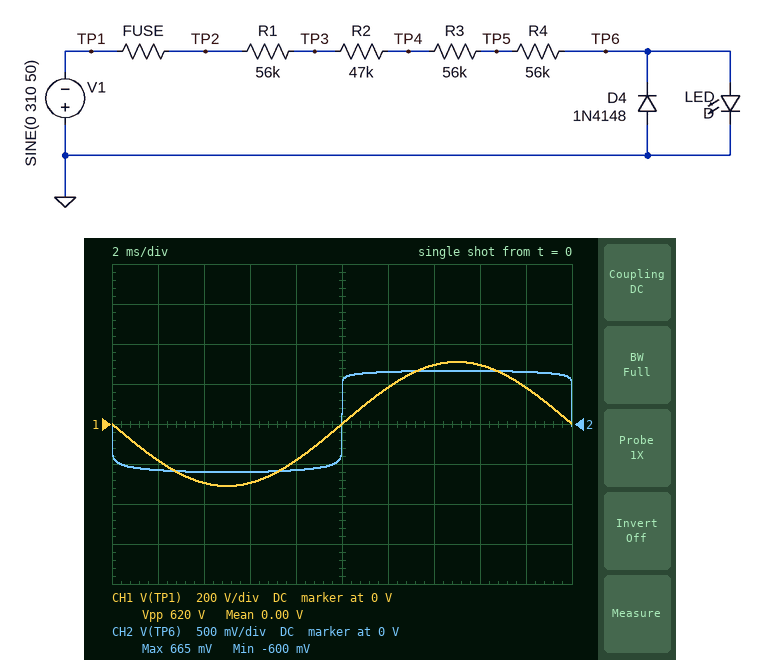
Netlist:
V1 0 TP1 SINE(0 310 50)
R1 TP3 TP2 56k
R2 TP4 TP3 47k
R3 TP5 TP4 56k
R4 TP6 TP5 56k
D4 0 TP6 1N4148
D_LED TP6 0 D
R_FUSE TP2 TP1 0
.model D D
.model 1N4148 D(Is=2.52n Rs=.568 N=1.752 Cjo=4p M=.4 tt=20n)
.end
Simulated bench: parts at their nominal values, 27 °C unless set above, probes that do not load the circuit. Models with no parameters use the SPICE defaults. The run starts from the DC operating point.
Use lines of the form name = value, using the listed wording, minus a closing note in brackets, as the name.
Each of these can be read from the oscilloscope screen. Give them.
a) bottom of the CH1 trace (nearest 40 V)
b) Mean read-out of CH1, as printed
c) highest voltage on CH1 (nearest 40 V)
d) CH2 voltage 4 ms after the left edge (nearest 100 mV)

bottom of the CH1 trace = -320 V
Mean read-out of CH1, as printed = 0.00 V
highest voltage on CH1 = 320 V
CH2 voltage 4 ms after the left edge = -600 mV
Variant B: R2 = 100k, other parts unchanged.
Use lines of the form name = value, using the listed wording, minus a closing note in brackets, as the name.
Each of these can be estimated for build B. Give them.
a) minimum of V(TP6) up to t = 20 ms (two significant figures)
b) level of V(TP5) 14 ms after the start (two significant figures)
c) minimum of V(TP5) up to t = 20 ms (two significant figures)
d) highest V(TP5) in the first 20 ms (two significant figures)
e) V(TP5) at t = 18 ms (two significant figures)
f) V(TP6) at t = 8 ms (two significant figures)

minimum of V(TP6) up to t = 20 ms = -590 mV
level of V(TP5) 14 ms after the start = 62 V
minimum of V(TP5) up to t = 20 ms = -65 V
highest V(TP5) in the first 20 ms = 65 V
V(TP5) at t = 18 ms = 39 V
V(TP6) at t = 8 ms = -570 mV
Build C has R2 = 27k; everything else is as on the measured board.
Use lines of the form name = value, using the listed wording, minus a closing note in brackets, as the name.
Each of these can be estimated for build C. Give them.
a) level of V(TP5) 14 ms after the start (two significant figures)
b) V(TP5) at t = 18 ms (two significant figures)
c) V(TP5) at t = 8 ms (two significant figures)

level of V(TP5) 14 ms after the start = 85 V
V(TP5) at t = 18 ms = 53 V
V(TP5) at t = 8 ms = -53 V
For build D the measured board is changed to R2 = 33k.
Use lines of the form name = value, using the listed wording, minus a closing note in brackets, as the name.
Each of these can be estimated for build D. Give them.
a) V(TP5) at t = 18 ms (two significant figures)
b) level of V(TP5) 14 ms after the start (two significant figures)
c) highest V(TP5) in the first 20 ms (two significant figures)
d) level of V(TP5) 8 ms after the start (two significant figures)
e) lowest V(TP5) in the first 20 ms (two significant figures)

V(TP5) at t = 18 ms = 51 V
level of V(TP5) 14 ms after the start = 83 V
highest V(TP5) in the first 20 ms = 87 V
level of V(TP5) 8 ms after the start = -51 V
lowest V(TP5) in the first 20 ms = -87 V
